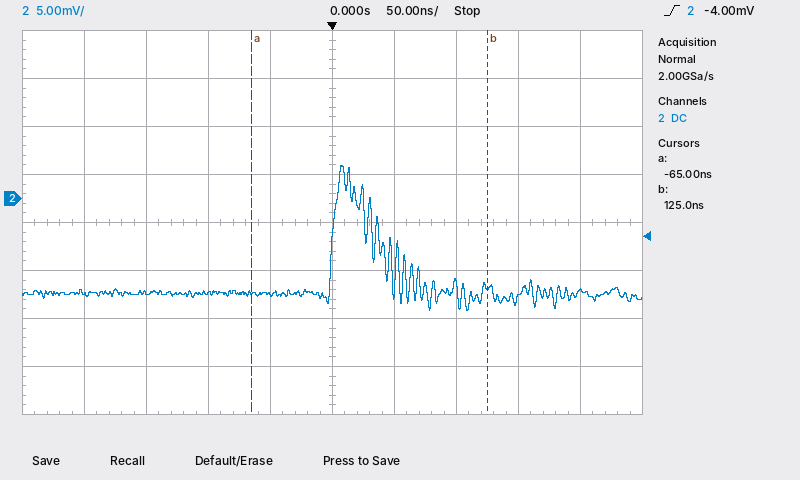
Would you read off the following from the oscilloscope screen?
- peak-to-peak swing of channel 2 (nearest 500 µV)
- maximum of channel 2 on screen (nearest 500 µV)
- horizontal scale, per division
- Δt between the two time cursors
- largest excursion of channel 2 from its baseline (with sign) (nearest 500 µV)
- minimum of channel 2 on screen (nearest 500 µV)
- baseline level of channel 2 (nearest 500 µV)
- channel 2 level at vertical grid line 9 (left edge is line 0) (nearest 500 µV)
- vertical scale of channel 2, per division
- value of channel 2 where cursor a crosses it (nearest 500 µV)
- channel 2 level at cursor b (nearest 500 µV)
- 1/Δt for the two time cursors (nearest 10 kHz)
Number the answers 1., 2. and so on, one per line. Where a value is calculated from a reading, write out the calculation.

1. 3.5 mV − (-11.5 mV) = 15.0 mV
2. 3.5 mV
3. 50 ns
4. 125 ns − (-65 ns) = 190 ns
5. 3.5 mV − (-10.0 mV) = +13.5 mV
6. -11.5 mV
7. -10.0 mV
8. -9.5 mV
9. 5 mV
10. -10.0 mV
11. -9.0 mV
12. 1 / 190 ns ≈ 5.26 MHz
